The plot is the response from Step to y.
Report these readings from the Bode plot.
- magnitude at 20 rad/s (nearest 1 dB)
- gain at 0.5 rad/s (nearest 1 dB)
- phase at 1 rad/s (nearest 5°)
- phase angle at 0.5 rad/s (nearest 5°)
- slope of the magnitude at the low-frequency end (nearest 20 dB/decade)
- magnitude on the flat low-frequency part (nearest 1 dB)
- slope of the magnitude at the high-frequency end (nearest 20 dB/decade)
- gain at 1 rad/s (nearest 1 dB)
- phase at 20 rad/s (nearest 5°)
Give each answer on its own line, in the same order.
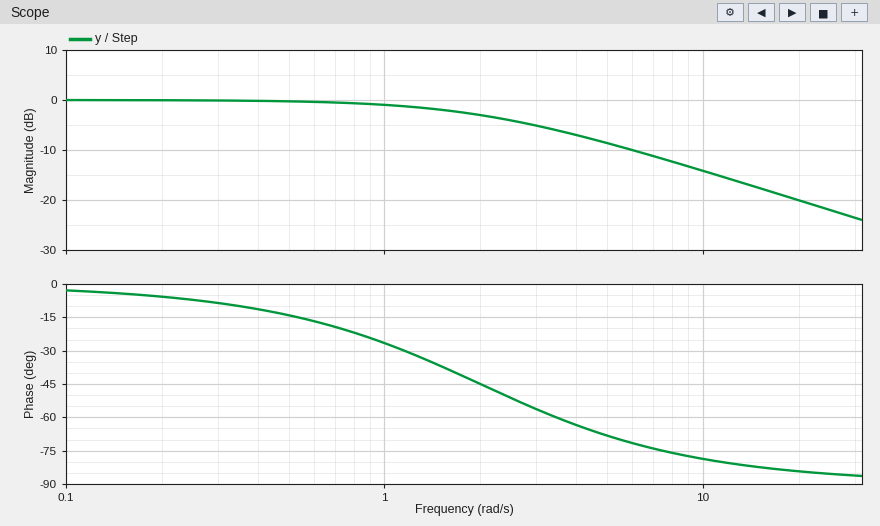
-20 dB
0 dB
-25°
-15°
0 dB/decade
0 dB
-20 dB/decade
-1 dB
-85°
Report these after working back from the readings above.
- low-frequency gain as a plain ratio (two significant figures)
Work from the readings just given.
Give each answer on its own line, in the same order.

1.0
